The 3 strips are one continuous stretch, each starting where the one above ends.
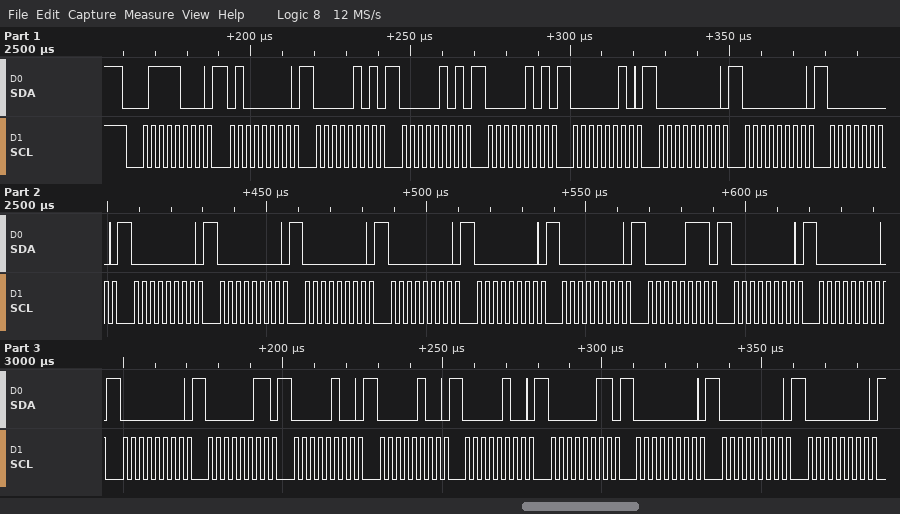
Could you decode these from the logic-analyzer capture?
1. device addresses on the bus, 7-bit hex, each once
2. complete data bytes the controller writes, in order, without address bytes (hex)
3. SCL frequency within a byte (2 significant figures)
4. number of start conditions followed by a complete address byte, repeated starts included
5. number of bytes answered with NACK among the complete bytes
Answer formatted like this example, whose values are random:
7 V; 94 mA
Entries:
0x3C; 40 05 05 05 02 00 00 00 00 00 00 00 00 00 07 00 00 00 03 04 04 04 03 00 00 00; 400 kHz; 1; 0
